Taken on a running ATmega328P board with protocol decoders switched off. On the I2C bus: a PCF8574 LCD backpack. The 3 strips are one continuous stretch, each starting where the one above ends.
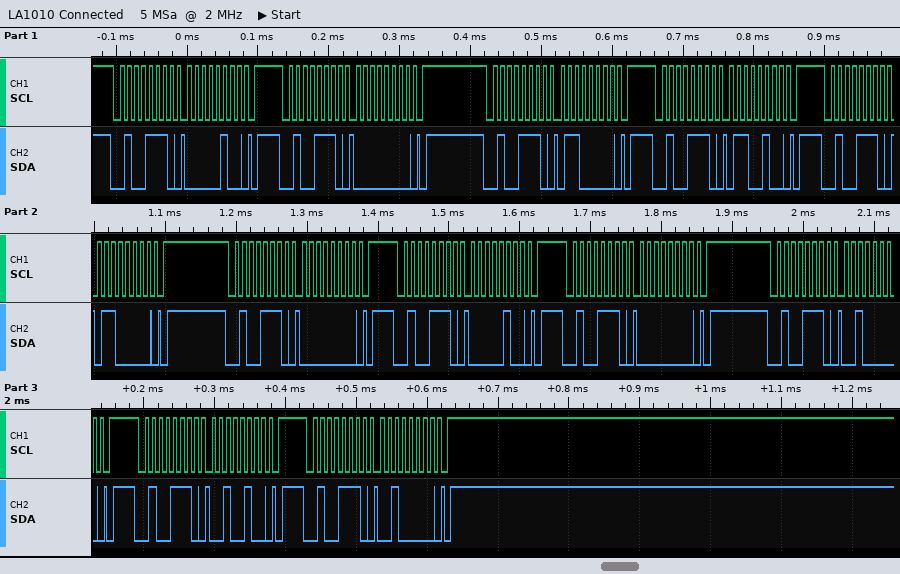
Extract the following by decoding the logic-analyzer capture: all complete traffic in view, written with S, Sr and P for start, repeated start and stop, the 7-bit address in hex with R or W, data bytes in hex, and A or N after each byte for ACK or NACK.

S 27W A 04 A P S 27W A 00 A P S 27W A 60 A P S 27W A 64 A P S 27W A 60 A P S 27W A 00 A P S 27W A 04 A P S 27W A 00 A P S 27W A 20 A P S 27W A 24 A P S 27W A 20 A P
